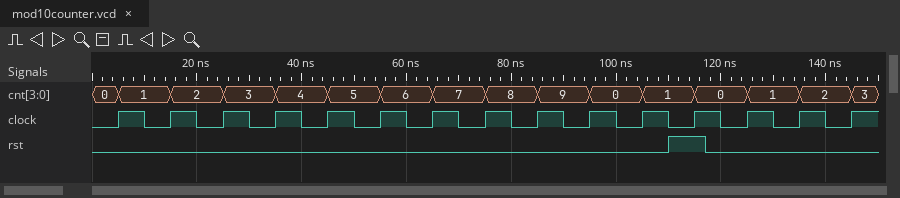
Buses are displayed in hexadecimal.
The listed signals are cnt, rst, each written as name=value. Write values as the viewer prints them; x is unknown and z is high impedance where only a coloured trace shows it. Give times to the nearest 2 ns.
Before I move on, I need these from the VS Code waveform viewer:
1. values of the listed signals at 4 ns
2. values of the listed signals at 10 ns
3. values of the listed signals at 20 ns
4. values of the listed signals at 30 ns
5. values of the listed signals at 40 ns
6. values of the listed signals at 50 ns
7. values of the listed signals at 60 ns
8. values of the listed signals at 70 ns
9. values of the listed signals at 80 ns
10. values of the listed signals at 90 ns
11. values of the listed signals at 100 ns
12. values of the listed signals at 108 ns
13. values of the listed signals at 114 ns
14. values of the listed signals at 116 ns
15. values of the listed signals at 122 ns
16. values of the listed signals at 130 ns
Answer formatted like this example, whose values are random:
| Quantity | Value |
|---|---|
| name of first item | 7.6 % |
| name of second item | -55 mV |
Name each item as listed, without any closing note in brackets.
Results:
| Quantity | Value |
|---|---|
| values of the listed signals at 4 ns | cnt=0, rst=0 |
| values of the listed signals at 10 ns | cnt=1, rst=0 |
| values of the listed signals at 20 ns | cnt=2, rst=0 |
| values of the listed signals at 30 ns | cnt=3, rst=0 |
| values of the listed signals at 40 ns | cnt=4, rst=0 |
| values of the listed signals at 50 ns | cnt=5, rst=0 |
| values of the listed signals at 60 ns | cnt=6, rst=0 |
| values of the listed signals at 70 ns | cnt=7, rst=0 |
| values of the listed signals at 80 ns | cnt=8, rst=0 |
| values of the listed signals at 90 ns | cnt=9, rst=0 |
| values of the listed signals at 100 ns | cnt=0, rst=0 |
| values of the listed signals at 108 ns | cnt=1, rst=0 |
| values of the listed signals at 114 ns | cnt=1, rst=1 |
| values of the listed signals at 116 ns | cnt=0, rst=1 |
| values of the listed signals at 122 ns | cnt=0, rst=0 |
| values of the listed signals at 130 ns | cnt=1, rst=0 |
